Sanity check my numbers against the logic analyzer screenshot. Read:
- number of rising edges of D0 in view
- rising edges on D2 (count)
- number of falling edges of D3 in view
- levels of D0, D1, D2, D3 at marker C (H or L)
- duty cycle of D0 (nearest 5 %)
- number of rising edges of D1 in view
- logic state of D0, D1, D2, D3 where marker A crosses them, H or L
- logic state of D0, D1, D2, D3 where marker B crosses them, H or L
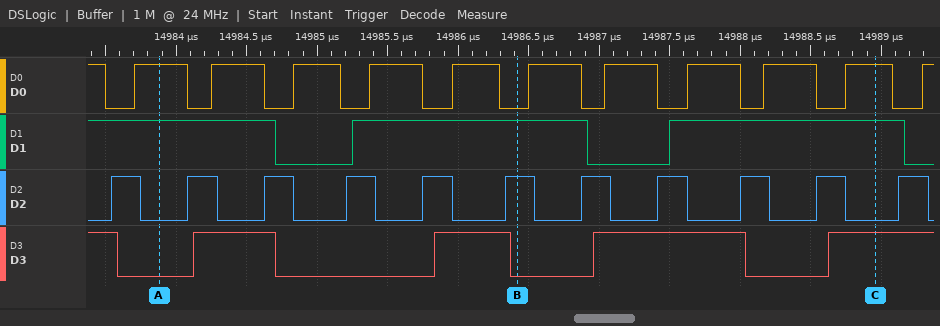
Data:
11
11
4
D0=H, D1=H, D2=L, D3=H
65 %
2
D0=H, D1=H, D2=L, D3=L
D0=L, D1=H, D2=H, D3=L
